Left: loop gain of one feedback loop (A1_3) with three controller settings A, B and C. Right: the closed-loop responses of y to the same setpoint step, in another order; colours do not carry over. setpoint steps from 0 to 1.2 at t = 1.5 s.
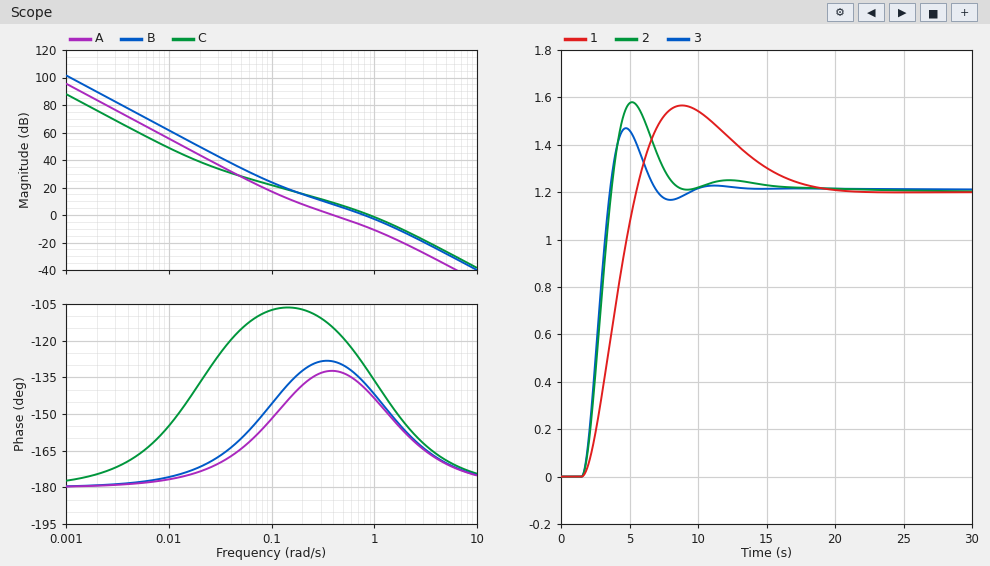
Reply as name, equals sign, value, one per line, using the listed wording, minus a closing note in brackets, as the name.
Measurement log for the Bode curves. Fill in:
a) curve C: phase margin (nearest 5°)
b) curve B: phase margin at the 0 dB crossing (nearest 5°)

curve C: phase margin = 45°
curve B: phase margin at the 0 dB crossing = 45°
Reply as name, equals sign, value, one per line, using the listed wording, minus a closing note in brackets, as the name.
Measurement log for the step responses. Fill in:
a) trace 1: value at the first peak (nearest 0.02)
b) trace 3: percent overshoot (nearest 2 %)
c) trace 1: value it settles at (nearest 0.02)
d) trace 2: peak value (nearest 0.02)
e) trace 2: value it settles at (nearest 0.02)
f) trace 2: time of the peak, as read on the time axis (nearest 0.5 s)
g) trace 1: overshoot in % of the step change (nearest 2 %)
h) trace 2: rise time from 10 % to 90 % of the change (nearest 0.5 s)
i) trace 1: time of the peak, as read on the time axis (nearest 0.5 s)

trace 1: value at the first peak = 1.56
trace 3: percent overshoot = 22 %
trace 1: value it settles at = 1.20
trace 2: peak value = 1.58
trace 2: value it settles at = 1.20
trace 2: time of the peak, as read on the time axis = 5.0 s
trace 1: overshoot in % of the step change = 30 %
trace 2: rise time from 10 % to 90 % of the change = 1.5 s
trace 1: time of the peak, as read on the time axis = 9.0 s
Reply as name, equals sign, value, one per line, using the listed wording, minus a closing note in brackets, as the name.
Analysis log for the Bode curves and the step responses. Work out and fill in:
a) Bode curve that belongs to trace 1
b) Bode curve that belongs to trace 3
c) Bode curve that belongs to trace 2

Bode curve that belongs to trace 1 = A
Bode curve that belongs to trace 3 = C
Bode curve that belongs to trace 2 = B
